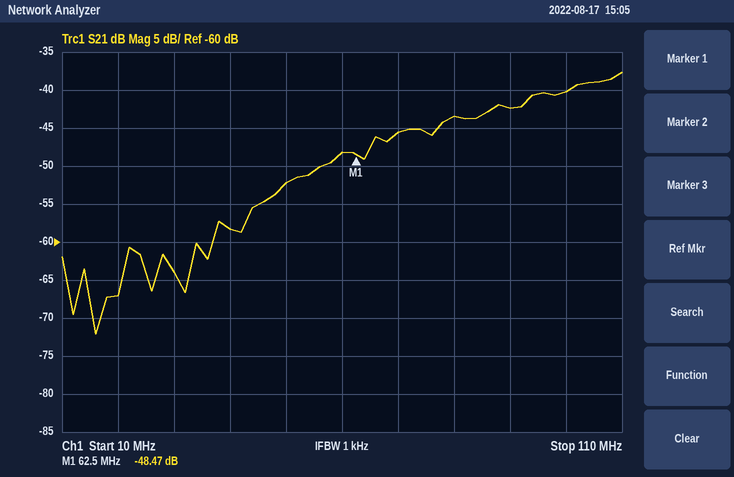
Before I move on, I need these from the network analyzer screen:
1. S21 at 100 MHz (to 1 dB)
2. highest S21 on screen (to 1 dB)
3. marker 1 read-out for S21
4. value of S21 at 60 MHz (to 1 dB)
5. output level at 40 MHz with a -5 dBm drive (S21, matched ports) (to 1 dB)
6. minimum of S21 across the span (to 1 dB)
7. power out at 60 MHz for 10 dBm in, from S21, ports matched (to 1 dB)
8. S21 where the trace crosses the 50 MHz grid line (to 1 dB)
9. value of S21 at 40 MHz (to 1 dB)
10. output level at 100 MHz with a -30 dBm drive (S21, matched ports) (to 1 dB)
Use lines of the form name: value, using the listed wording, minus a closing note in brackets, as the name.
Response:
S21 at 100 MHz: -40 dB
highest S21 on screen: -38 dB
marker 1 read-out for S21: -48.47 dB
value of S21 at 60 MHz: -48 dB
output level at 40 MHz with a -5 dBm drive (S21, matched ports): -63 dBm
minimum of S21 across the span: -72 dB
power out at 60 MHz for 10 dBm in, from S21, ports matched: -38 dBm
S21 where the trace crosses the 50 MHz grid line: -52 dB
value of S21 at 40 MHz: -58 dB
output level at 100 MHz with a -30 dBm drive (S21, matched ports): -70 dBm
